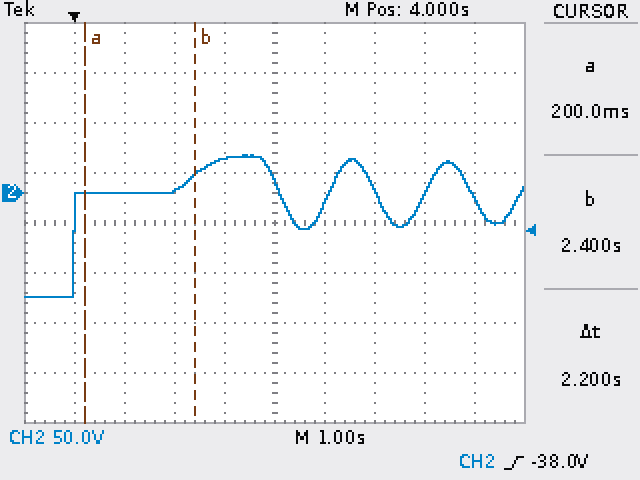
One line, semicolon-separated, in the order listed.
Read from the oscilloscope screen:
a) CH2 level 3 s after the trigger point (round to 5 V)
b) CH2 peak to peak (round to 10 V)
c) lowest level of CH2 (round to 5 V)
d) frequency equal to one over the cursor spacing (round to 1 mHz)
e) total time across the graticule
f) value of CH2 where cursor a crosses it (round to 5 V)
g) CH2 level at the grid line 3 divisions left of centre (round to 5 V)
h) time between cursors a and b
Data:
35 V; 140 V; -105 V; 455 mHz; 10 s; 0 V; 0 V; 2.2 s
